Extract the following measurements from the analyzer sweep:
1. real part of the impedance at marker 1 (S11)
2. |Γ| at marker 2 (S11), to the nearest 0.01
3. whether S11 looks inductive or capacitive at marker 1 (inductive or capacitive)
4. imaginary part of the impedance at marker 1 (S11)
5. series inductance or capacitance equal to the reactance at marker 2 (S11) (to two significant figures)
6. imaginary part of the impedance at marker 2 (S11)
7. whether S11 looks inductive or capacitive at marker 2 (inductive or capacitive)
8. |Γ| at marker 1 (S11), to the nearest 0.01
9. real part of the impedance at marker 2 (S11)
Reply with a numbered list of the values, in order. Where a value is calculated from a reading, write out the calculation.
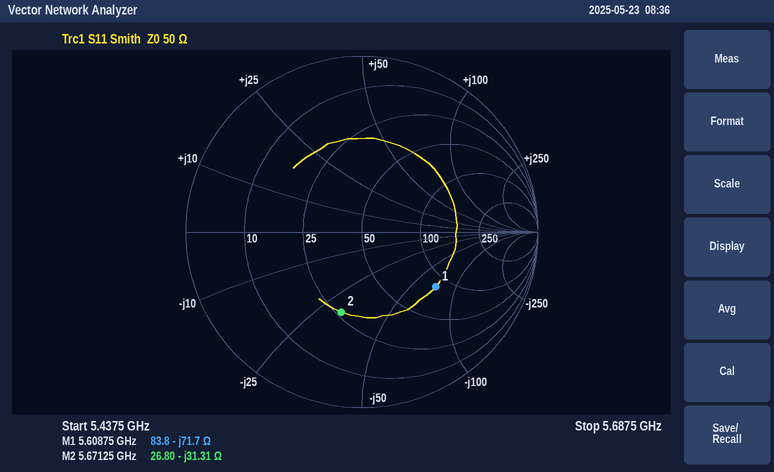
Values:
1. 83.8 Ω
2. 0.47
3. capacitive
4. -71.7 Ω
5. C = 1/(2π × 5.67125 GHz × 31.31 Ω) ≈ 896 fF, so 900 fF to two significant figures
6. -31.31 Ω
7. capacitive
8. 0.52
9. 26.80 Ω
